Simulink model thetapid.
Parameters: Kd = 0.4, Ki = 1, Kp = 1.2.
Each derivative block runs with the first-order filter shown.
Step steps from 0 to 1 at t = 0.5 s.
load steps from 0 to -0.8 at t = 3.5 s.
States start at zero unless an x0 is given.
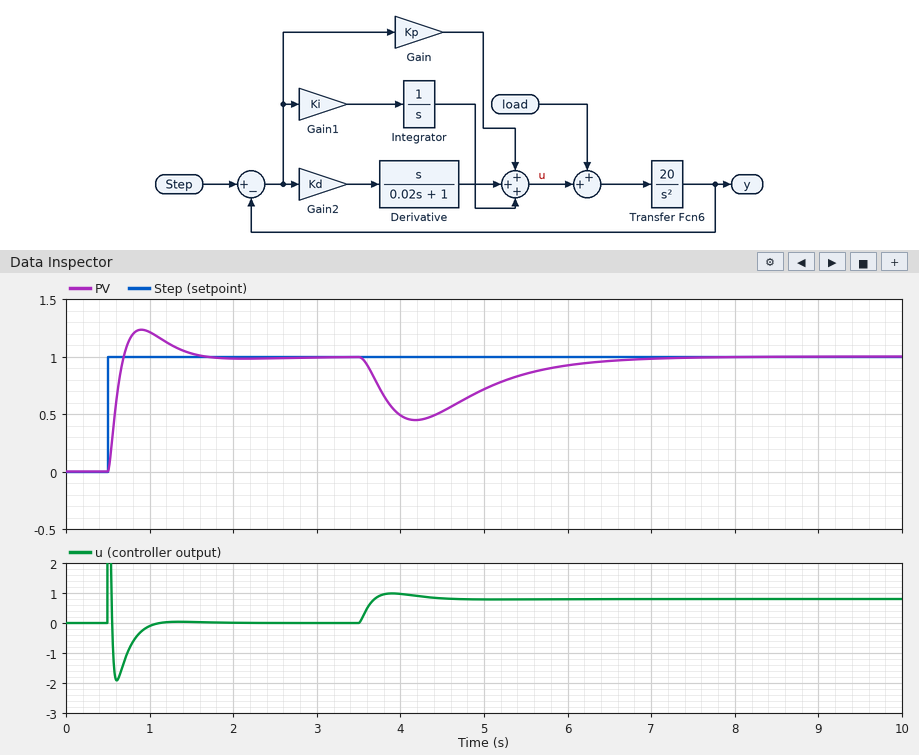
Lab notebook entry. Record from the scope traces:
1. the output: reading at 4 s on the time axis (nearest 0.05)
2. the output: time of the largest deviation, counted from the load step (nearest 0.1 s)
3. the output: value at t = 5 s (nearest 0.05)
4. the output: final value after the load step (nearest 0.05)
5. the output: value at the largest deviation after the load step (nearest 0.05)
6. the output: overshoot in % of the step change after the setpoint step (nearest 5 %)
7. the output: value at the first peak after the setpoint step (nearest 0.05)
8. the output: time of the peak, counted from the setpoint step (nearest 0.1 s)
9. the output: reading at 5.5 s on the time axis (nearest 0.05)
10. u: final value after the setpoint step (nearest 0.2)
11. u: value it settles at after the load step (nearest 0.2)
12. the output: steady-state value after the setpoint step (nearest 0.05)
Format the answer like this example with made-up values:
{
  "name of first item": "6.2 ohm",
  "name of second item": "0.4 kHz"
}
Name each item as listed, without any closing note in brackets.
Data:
{
  "the output: reading at 4 s on the time axis": "0.50",
  "the output: time of the largest deviation, counted from the load step": "0.7 s",
  "the output: value at t = 5 s": "0.70",
  "the output: final value after the load step": "1.00",
  "the output: value at the largest deviation after the load step": "0.45",
  "the output: overshoot in % of the step change after the setpoint step": "25 %",
  "the output: value at the first peak after the setpoint step": "1.25",
  "the output: time of the peak, counted from the setpoint step": "0.4 s",
  "the output: reading at 5.5 s on the time axis": "0.85",
  "u: final value after the setpoint step": "0.0",
  "u: value it settles at after the load step": "0.8",
  "the output: steady-state value after the setpoint step": "1.00"
}
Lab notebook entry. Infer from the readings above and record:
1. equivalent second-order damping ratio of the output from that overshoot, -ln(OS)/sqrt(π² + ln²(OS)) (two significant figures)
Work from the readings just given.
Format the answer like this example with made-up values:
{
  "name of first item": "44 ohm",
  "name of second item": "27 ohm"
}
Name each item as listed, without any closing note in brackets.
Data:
{
  "equivalent second-order damping ratio of the output from that overshoot, -ln(OS)/sqrt(π² + ln²(OS))": "0.40"
}
